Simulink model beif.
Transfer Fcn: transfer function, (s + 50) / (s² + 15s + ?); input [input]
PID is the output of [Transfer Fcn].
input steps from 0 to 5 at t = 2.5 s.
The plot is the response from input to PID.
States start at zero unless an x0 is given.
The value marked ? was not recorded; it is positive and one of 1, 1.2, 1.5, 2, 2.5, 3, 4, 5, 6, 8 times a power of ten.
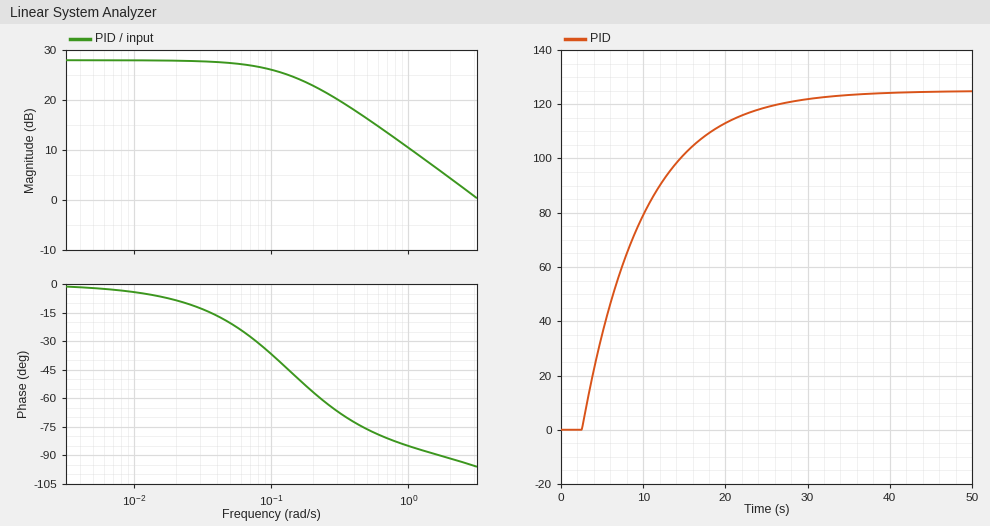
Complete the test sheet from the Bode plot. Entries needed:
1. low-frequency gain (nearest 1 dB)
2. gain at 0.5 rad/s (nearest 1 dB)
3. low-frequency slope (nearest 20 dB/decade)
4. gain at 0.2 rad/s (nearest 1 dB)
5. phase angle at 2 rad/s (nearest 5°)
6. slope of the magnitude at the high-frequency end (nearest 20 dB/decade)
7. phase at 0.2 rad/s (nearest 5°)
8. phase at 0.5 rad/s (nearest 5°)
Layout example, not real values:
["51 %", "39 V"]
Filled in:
["28 dB", "16 dB", "0 dB/decade", "23 dB", "-90°", "-20 dB/decade", "-55°", "-75°"]
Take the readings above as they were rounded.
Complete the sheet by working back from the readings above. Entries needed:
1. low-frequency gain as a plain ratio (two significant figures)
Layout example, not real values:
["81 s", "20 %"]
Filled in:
["25"]
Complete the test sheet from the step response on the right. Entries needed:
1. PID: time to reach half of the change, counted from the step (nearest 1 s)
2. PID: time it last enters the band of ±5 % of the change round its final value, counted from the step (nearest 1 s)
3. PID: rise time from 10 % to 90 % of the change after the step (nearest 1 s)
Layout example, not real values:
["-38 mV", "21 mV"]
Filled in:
["5 s", "22 s", "16 s"]
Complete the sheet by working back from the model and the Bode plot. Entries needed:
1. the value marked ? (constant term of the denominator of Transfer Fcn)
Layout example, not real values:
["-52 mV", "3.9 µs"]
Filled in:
["2"]
